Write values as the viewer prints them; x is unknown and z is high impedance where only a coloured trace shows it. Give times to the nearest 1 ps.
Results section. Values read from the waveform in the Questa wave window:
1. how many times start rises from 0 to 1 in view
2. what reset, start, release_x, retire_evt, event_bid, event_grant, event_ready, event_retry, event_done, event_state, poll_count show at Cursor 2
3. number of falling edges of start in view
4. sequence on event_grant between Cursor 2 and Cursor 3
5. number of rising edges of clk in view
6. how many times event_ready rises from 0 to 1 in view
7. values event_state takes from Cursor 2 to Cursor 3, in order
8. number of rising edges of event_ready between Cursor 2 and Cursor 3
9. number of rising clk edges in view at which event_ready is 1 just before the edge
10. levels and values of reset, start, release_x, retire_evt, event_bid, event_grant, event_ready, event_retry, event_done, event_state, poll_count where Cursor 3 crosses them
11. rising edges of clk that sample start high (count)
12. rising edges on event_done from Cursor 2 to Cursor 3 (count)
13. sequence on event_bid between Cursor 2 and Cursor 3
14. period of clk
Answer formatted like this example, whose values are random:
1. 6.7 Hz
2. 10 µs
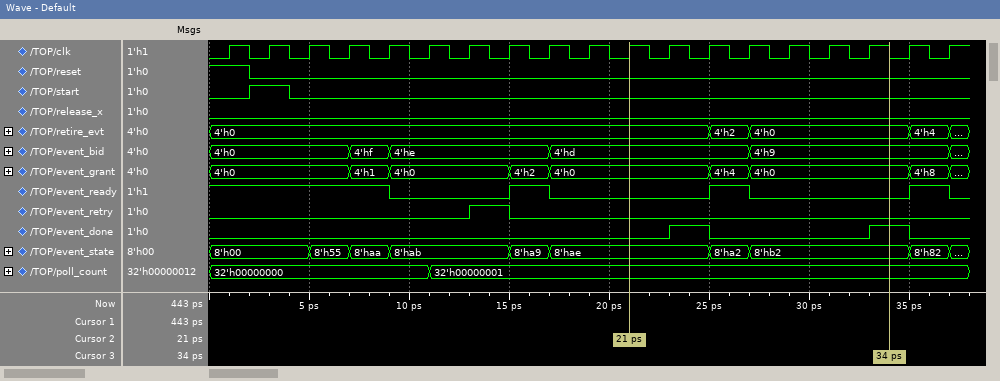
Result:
1. 1
2. reset=0, start=0, release_x=0, retire_evt=4'h0, event_bid=4'hd, event_grant=4'h0, event_ready=0, event_retry=0, event_done=0, event_state=8'hae, poll_count=32'h00000001
3. 1
4. 4'h0, 4'h4, 4'h0
5. 19
6. 3
7. 8'hae, 8'ha2, 8'hb2
8. 1
9. 8
10. reset=0, start=0, release_x=0, retire_evt=4'h0, event_bid=4'h9, event_grant=4'h0, event_ready=0, event_retry=0, event_done=1, event_state=8'hb2, poll_count=32'h00000001
11. 1
12. 2
13. 4'hd, 4'h9
14. 2 ps
